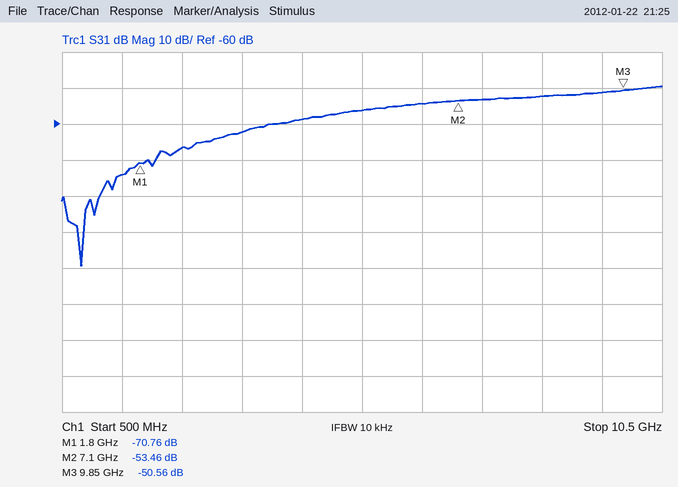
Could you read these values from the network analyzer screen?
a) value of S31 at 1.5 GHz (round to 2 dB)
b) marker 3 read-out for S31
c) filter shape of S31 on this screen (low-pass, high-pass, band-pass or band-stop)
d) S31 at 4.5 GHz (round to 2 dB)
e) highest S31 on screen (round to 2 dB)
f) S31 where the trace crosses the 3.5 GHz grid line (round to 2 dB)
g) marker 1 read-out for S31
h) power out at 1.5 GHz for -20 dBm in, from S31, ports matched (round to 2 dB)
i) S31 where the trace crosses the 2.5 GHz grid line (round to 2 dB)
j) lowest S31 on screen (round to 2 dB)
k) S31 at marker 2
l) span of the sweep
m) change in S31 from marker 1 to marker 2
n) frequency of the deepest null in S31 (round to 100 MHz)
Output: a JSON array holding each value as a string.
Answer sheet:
["-74 dB", "-50.56 dB", "high-pass", "-58 dB", "-50 dB", "-62 dB", "-70.76 dB", "-94 dBm", "-66 dB", "-100 dB", "-53.46 dB", "10 GHz", "17.30 dB", "800 MHz"]
